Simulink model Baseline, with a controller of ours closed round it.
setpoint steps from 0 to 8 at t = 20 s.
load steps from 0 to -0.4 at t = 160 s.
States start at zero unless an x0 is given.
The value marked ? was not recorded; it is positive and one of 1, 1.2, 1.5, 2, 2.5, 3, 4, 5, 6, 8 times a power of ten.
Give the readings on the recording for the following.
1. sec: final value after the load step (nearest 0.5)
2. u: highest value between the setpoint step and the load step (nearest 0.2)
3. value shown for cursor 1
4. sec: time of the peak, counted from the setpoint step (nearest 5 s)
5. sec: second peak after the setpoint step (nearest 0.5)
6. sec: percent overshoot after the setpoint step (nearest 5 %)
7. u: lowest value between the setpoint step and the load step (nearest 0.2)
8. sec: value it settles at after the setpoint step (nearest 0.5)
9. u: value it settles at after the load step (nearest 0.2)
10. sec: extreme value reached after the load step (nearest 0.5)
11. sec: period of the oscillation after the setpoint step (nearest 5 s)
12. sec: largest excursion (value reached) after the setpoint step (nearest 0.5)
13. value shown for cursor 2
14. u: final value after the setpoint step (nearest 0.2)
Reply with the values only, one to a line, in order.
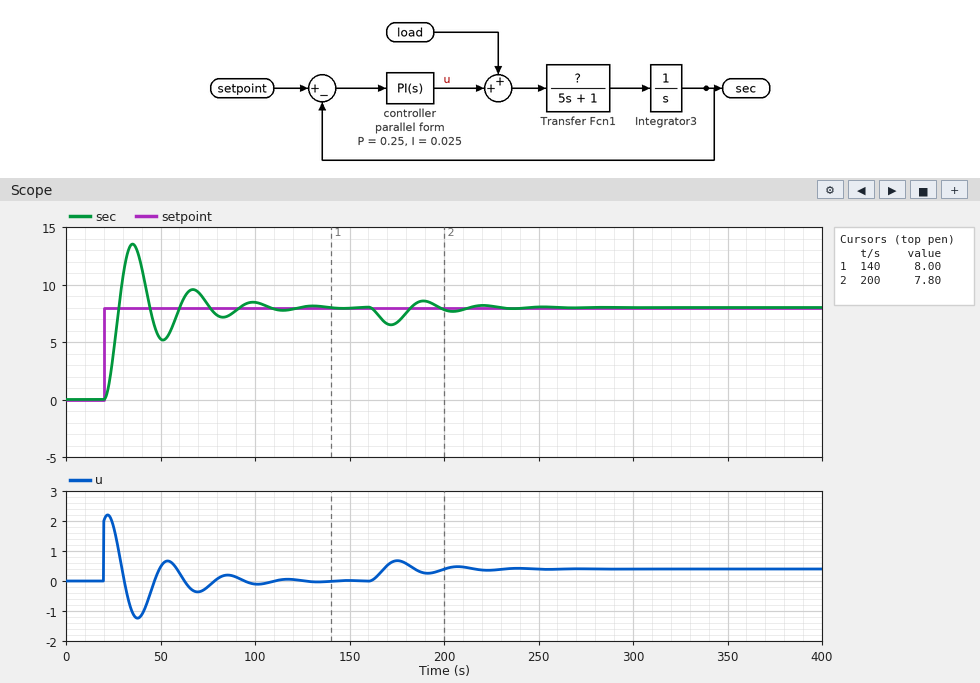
8.0
2.2
8.00
15 s
9.5
70 %
-1.2
8.0
0.4
6.5
30 s
13.5
7.80
0.0
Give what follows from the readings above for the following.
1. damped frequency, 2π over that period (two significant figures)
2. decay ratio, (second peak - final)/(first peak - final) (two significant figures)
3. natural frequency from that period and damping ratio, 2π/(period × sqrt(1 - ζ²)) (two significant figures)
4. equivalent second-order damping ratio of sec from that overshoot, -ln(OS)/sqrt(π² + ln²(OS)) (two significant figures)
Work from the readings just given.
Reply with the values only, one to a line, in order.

0.21 rad/s
0.27
0.21 rad/s
0.11
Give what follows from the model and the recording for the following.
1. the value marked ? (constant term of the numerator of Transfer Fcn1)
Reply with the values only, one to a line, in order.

1
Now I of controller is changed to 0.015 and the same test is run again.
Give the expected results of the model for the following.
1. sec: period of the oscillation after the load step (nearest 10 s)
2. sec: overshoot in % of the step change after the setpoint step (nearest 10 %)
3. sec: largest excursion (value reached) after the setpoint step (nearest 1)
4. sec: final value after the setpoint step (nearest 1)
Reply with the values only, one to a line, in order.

30 s
50 %
12
8
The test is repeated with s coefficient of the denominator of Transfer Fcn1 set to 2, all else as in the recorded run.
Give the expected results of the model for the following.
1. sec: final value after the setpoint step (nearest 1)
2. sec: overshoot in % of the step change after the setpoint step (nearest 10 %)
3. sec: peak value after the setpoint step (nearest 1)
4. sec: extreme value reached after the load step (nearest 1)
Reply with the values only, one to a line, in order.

8
40 %
11
7
